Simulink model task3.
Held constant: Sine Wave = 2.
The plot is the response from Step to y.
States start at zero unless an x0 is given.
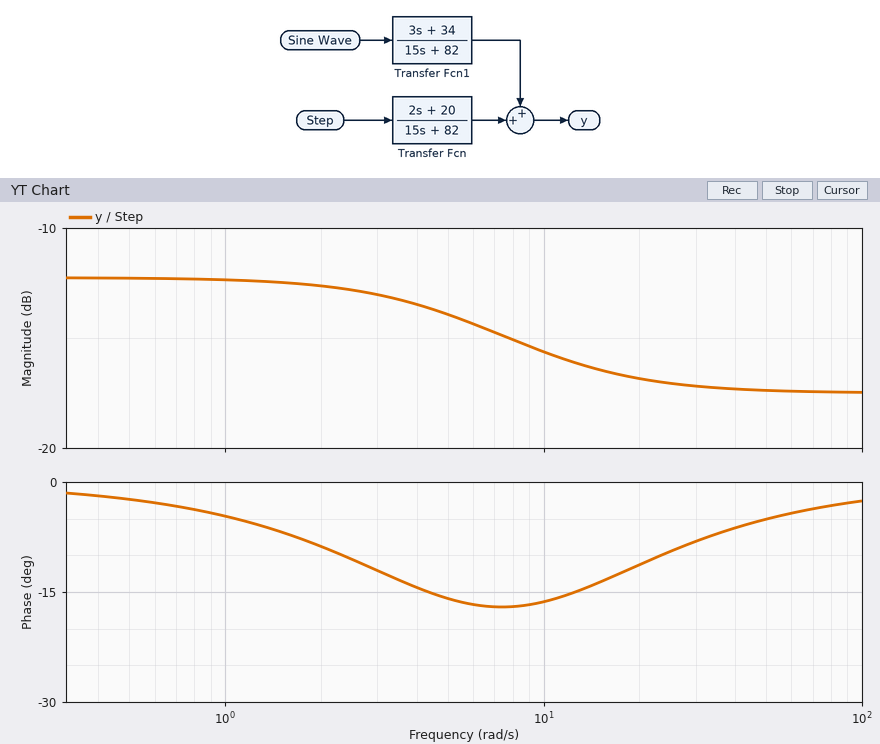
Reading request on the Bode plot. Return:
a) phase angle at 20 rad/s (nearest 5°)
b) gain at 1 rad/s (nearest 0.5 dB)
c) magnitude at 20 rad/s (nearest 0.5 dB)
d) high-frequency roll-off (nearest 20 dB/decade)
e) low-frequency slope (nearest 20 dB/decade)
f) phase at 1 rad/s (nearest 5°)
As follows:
-10°
-12.5 dB
-17.0 dB
0 dB/decade
0 dB/decade
-5°
